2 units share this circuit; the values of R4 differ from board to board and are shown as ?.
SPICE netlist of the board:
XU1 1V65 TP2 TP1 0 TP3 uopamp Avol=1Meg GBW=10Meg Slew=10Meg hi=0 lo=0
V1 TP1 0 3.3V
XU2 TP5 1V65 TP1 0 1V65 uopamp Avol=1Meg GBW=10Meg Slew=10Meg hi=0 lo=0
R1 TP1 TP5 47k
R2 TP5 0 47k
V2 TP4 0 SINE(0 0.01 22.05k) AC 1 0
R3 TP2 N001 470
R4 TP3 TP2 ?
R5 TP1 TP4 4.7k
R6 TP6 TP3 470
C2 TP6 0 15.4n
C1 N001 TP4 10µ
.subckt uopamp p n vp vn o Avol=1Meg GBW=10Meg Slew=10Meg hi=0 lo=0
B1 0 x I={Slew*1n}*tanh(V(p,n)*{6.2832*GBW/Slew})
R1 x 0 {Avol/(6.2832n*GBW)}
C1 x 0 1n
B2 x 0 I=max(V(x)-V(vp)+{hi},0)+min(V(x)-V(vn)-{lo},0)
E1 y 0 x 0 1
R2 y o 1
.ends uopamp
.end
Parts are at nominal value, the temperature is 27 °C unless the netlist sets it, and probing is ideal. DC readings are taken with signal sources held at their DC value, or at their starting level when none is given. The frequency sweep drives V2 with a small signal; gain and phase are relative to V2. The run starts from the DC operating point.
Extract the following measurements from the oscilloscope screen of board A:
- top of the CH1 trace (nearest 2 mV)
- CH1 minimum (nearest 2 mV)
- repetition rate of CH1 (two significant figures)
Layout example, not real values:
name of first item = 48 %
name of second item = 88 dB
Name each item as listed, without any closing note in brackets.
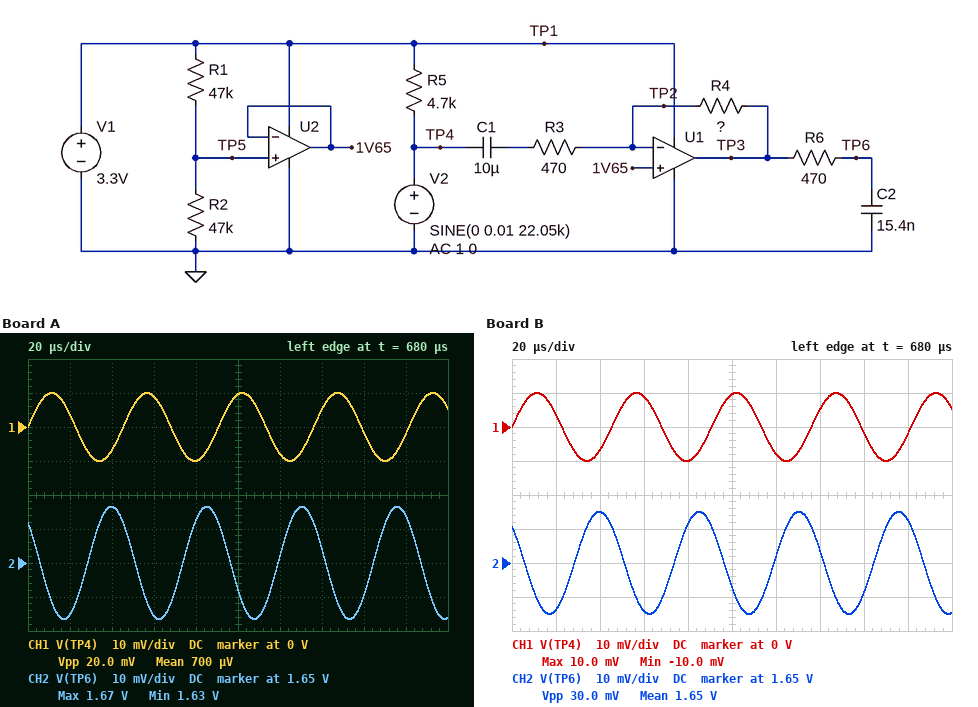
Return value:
top of the CH1 trace = 10 mV
CH1 minimum = -10 mV
repetition rate of CH1 = 22 kHz
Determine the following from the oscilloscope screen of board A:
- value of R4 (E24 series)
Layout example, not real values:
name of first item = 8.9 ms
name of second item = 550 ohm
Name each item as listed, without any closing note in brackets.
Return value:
value of R4 = 1.1 kΩ
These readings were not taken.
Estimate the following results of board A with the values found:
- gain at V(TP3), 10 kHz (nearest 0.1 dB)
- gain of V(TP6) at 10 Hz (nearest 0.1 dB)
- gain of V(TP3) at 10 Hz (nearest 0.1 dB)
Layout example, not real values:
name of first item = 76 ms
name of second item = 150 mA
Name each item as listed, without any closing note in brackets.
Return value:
gain at V(TP3), 10 kHz = 7.4 dB
gain of V(TP6) at 10 Hz = -3.6 dB
gain of V(TP3) at 10 Hz = -3.6 dB
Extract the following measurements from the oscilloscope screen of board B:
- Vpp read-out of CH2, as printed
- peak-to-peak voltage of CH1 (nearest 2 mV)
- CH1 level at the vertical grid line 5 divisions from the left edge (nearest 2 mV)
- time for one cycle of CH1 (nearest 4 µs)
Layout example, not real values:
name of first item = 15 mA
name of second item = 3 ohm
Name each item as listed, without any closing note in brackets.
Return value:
Vpp read-out of CH2, as printed = 30.0 mV
peak-to-peak voltage of CH1 = 20 mV
CH1 level at the vertical grid line 5 divisions from the left edge = 10 mV
time for one cycle of CH1 = 44 µs
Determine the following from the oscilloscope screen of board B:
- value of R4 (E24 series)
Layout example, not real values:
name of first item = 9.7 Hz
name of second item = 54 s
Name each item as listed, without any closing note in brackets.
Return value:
value of R4 = 1 kΩ
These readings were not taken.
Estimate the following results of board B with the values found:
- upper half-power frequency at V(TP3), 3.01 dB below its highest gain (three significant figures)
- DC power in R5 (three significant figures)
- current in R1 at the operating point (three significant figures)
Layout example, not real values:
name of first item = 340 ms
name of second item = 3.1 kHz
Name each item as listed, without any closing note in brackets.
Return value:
upper half-power frequency at V(TP3), 3.01 dB below its highest gain = 3.19 MHz
DC power in R5 = 2.32 mW
current in R1 at the operating point = 35.1 µA
